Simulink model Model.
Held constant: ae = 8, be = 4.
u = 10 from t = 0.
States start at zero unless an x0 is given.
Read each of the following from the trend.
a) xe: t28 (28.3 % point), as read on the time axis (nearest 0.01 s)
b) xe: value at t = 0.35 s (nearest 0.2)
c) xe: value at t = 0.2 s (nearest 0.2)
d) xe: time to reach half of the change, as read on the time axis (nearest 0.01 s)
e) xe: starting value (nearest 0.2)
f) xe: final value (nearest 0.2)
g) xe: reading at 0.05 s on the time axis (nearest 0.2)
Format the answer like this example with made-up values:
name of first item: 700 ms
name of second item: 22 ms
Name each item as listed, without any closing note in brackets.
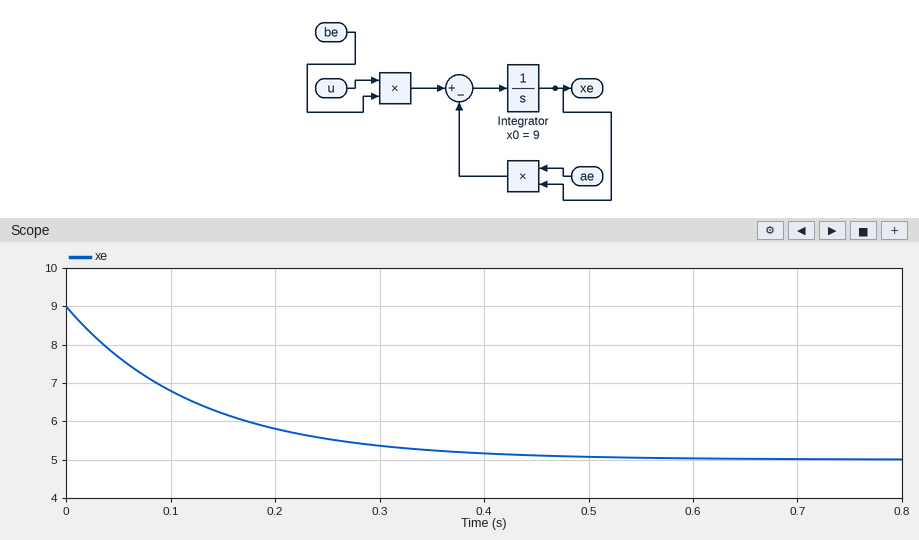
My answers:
xe: t28 (28.3 % point), as read on the time axis: 0.04 s
xe: value at t = 0.35 s: 5.2
xe: value at t = 0.2 s: 5.8
xe: time to reach half of the change, as read on the time axis: 0.09 s
xe: starting value: 9.0
xe: final value: 5.0
xe: reading at 0.05 s on the time axis: 7.6
